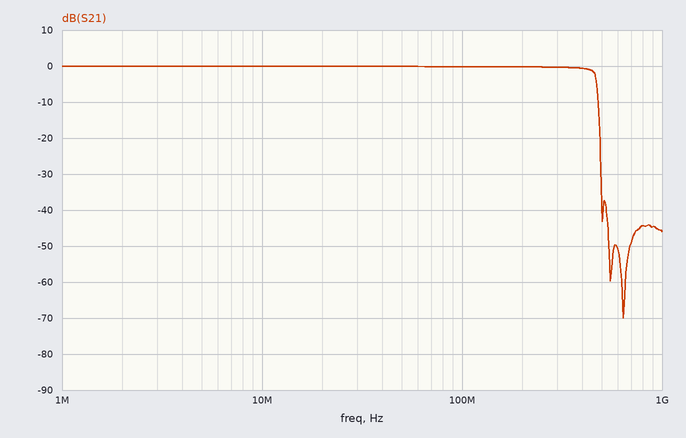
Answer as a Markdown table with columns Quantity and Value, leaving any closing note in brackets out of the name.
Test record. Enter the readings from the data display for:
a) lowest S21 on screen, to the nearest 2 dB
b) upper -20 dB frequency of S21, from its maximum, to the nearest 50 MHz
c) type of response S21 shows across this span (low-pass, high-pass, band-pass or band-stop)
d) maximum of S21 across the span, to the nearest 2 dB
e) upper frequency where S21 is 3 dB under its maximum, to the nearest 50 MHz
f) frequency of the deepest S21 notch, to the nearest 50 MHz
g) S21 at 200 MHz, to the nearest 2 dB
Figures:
| Quantity | Value |
|---|---|
| lowest S21 on screen, to the nearest 2 dB | -70 dB |
| upper -20 dB frequency of S21, from its maximum, to the nearest 50 MHz | 500 MHz |
| type of response S21 shows across this span | low-pass |
| maximum of S21 across the span, to the nearest 2 dB | 0 dB |
| upper frequency where S21 is 3 dB under its maximum, to the nearest 50 MHz | 450 MHz |
| frequency of the deepest S21 notch, to the nearest 50 MHz | 650 MHz |
| S21 at 200 MHz, to the nearest 2 dB | 0 dB |
